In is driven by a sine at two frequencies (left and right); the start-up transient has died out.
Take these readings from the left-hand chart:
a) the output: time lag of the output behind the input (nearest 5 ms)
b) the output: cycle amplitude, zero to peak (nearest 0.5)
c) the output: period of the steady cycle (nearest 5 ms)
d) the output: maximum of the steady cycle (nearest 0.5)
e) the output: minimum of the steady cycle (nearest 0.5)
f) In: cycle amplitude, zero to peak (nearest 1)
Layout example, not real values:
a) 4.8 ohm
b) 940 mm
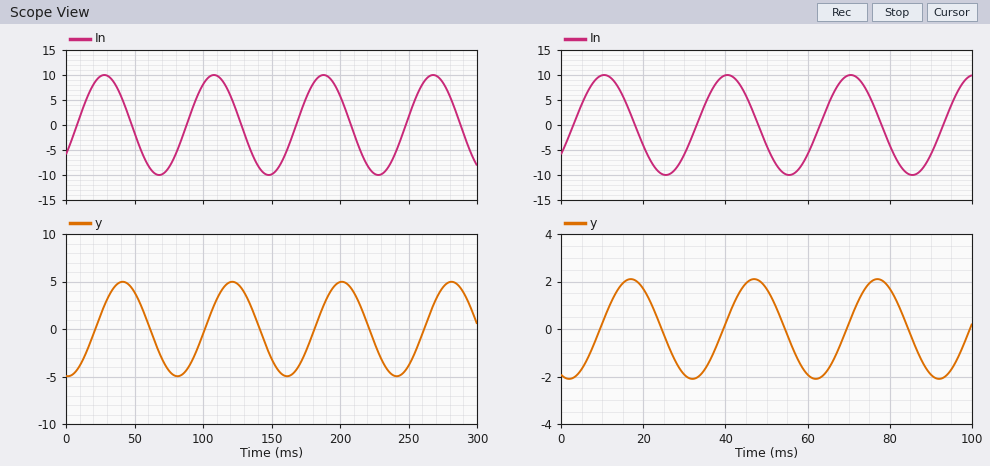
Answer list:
a) 15 ms
b) 5.0
c) 80 ms
d) 5.0
e) -5.0
f) 10
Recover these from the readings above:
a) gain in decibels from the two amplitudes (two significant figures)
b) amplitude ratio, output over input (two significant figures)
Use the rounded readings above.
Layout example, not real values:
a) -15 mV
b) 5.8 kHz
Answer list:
a) -6.0 dB
b) 0.50
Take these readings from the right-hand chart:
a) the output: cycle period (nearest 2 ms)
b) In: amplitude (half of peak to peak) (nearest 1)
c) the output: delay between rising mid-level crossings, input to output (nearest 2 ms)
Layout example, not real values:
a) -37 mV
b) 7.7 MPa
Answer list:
a) 30 ms
b) 10
c) 6 ms
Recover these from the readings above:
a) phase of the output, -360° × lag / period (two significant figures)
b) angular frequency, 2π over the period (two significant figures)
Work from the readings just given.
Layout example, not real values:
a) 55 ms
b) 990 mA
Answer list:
a) -72°
b) 0.21 rad/ms
